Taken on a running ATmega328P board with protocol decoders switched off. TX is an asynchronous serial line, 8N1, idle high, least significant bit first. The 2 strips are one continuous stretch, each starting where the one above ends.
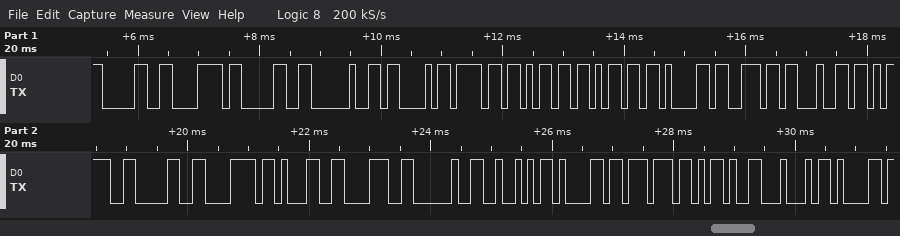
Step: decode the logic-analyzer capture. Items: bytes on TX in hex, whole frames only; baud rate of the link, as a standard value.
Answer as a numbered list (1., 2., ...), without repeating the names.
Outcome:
1. 30 78 30 20 43 6F 6D 6D 61 6E 64 3D 30 78 31 38 20 52 61 77 2D 44 61
2. 9600 baud
